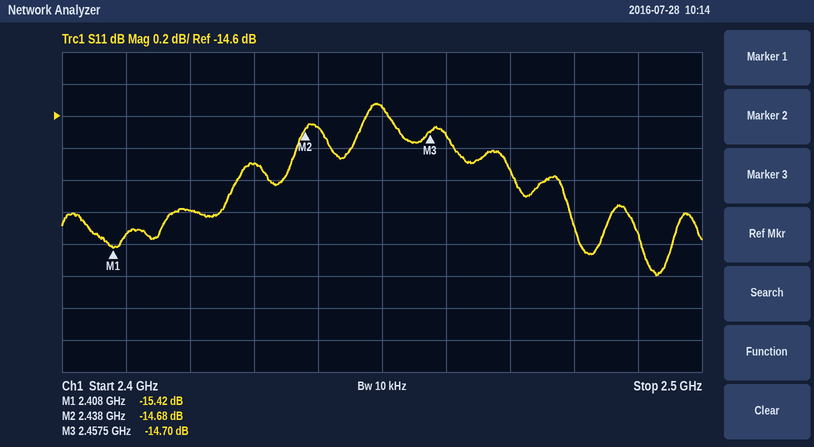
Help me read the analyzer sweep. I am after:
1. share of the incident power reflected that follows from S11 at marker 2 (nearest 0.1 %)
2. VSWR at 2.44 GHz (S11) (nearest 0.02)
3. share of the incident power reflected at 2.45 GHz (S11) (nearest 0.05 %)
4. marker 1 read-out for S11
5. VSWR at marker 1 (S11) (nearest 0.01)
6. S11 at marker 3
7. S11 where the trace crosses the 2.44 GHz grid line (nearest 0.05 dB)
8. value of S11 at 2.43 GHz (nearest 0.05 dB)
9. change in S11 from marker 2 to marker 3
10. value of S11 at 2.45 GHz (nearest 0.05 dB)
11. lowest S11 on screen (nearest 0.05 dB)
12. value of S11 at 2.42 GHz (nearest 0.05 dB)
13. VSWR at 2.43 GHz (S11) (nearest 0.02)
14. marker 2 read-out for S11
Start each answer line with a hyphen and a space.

- 3.4 %
- 1.46
- 3.50 %
- -15.42 dB
- 1.41
- -14.70 dB
- -14.65 dB
- -14.90 dB
- -0.02 dB
- -14.55 dB
- -15.60 dB
- -15.20 dB
- 1.44
- -14.68 dB
